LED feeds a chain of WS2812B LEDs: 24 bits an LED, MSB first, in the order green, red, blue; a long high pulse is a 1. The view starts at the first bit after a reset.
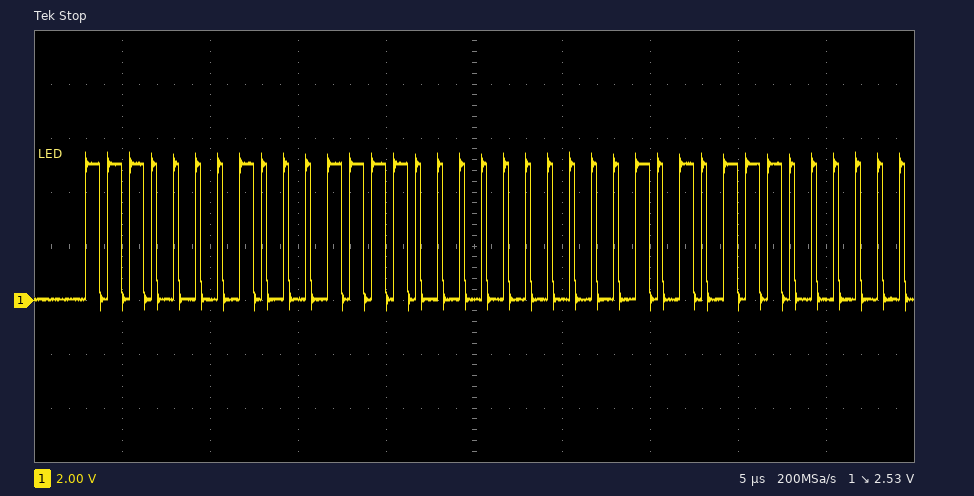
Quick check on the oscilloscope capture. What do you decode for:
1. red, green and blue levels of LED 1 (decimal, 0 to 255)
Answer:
30, 225, 0
